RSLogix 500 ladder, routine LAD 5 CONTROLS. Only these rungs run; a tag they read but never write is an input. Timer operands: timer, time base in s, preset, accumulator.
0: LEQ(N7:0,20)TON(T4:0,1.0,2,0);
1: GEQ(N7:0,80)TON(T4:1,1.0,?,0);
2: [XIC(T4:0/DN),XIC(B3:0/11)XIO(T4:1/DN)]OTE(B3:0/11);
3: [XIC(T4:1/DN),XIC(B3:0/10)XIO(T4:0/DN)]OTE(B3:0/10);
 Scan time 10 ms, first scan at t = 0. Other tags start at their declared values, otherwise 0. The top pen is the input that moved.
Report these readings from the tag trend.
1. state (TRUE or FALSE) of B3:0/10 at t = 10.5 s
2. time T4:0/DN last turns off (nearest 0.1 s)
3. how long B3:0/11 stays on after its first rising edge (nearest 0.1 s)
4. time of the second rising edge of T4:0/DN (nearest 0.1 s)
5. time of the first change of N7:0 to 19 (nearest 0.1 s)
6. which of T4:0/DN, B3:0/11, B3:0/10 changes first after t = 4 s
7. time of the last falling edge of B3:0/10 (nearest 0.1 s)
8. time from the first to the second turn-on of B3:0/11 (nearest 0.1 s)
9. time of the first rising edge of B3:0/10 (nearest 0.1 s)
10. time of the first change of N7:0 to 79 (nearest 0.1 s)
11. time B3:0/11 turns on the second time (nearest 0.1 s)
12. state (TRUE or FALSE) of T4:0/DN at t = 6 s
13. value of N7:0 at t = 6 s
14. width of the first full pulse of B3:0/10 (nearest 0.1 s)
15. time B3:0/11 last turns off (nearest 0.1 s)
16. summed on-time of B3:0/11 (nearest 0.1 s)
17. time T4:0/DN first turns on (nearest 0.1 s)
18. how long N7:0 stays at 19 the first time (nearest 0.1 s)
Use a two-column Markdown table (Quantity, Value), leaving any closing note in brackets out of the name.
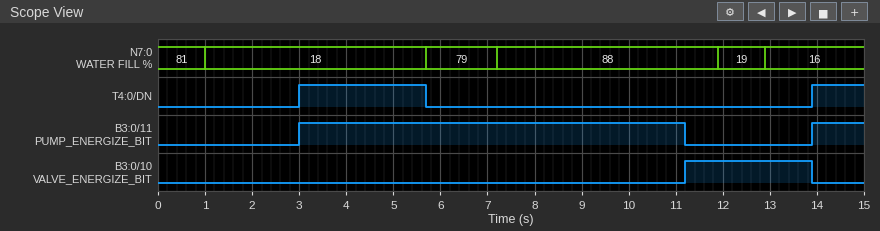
| Quantity | Value |
|---|---|
| state (TRUE or FALSE) of B3:0/10 at t = 10.5 s | FALSE |
| time T4:0/DN last turns off | 5.7 s |
| how long B3:0/11 stays on after its first rising edge | 8.2 s |
| time of the second rising edge of T4:0/DN | 13.9 s |
| time of the first change of N7:0 to 19 | 11.9 s |
| which of T4:0/DN, B3:0/11, B3:0/10 changes first after t = 4 s | T4:0/DN |
| time of the last falling edge of B3:0/10 | 13.9 s |
| time from the first to the second turn-on of B3:0/11 | 10.9 s |
| time of the first rising edge of B3:0/10 | 11.2 s |
| time of the first change of N7:0 to 79 | 5.7 s |
| time B3:0/11 turns on the second time | 13.9 s |
| state (TRUE or FALSE) of T4:0/DN at t = 6 s | FALSE |
| value of N7:0 at t = 6 s | 79 |
| width of the first full pulse of B3:0/10 | 2.7 s |
| time B3:0/11 last turns off | 11.2 s |
| summed on-time of B3:0/11 | 9.3 s |
| time T4:0/DN first turns on | 3.0 s |
| how long N7:0 stays at 19 the first time | 1.0 s |
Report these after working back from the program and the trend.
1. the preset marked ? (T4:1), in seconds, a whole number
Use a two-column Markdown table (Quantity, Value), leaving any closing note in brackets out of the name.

| Quantity | Value |
|---|---|
| the preset marked ? (T4:1), in seconds, a whole number | 4 s |
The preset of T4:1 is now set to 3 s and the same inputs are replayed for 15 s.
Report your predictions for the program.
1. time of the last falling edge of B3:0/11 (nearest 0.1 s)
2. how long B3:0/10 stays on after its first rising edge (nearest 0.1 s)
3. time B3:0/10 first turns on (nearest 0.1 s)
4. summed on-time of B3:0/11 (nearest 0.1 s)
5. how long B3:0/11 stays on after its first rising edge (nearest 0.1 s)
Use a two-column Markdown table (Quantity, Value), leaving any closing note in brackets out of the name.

| Quantity | Value |
|---|---|
| time of the last falling edge of B3:0/11 | 10.2 s |
| how long B3:0/10 stays on after its first rising edge | 3.7 s |
| time B3:0/10 first turns on | 10.2 s |
| summed on-time of B3:0/11 | 8.3 s |
| how long B3:0/11 stays on after its first rising edge | 7.2 s |
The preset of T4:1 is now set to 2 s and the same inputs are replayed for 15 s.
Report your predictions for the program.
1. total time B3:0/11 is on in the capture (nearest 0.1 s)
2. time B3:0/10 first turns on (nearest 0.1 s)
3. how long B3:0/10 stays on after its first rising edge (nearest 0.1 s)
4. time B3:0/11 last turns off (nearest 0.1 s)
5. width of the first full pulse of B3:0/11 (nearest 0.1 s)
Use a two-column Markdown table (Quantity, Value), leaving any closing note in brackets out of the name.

| Quantity | Value |
|---|---|
| total time B3:0/11 is on in the capture | 7.3 s |
| time B3:0/10 first turns on | 9.2 s |
| how long B3:0/10 stays on after its first rising edge | 4.7 s |
| time B3:0/11 last turns off | 9.2 s |
| width of the first full pulse of B3:0/11 | 6.2 s |
